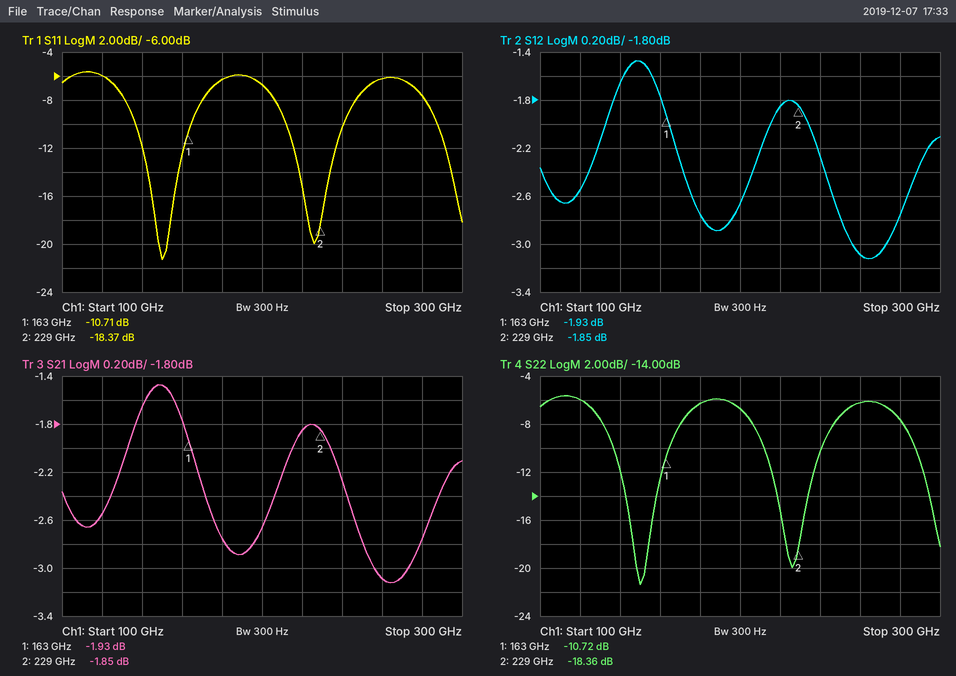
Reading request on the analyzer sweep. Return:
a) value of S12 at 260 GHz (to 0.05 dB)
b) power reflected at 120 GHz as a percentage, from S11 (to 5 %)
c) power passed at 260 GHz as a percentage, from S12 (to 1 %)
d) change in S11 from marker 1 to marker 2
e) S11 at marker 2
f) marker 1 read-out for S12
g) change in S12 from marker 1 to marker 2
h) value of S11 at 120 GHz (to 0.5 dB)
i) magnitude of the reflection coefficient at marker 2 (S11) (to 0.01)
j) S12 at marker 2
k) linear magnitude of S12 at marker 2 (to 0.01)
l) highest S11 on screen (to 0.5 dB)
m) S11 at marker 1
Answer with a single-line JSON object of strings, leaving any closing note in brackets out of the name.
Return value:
{"value of S12 at 260 GHz": "-3.10 dB", "power reflected at 120 GHz as a percentage, from S11": "25 %", "power passed at 260 GHz as a percentage, from S12": "49 %", "change in S11 from marker 1 to marker 2": "-7.66 dB", "S11 at marker 2": "-18.37 dB", "marker 1 read-out for S12": "-1.93 dB", "change in S12 from marker 1 to marker 2": "0.08 dB", "value of S11 at 120 GHz": "-6.0 dB", "magnitude of the reflection coefficient at marker 2 (S11)": "0.12", "S12 at marker 2": "-1.85 dB", "linear magnitude of S12 at marker 2": "0.81", "highest S11 on screen": "-5.5 dB", "S11 at marker 1": "-10.71 dB"}
